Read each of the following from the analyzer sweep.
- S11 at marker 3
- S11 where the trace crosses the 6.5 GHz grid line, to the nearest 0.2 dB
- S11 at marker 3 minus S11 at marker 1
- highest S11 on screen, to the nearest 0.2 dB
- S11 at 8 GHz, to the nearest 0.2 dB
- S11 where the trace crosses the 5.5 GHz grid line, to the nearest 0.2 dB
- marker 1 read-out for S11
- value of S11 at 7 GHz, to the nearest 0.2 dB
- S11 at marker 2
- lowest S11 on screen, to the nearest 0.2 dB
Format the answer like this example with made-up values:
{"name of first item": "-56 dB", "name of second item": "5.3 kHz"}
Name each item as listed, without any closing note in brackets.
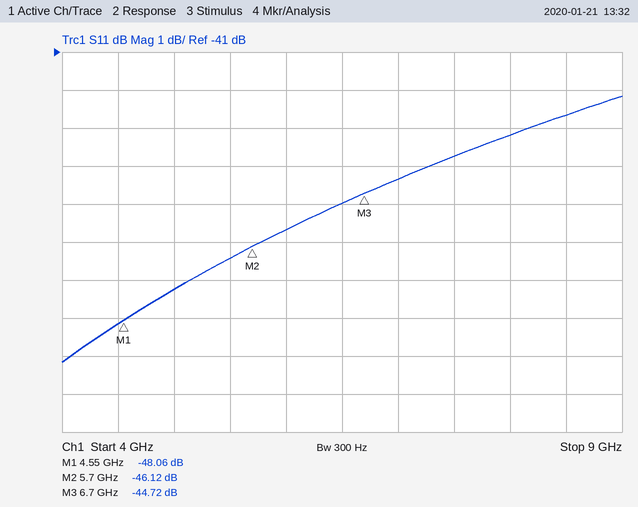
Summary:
{"S11 at marker 3": "-44.72 dB", "S11 where the trace crosses the 6.5 GHz grid line, to the nearest 0.2 dB": "-45.0 dB", "S11 at marker 3 minus S11 at marker 1": "3.34 dB", "highest S11 on screen, to the nearest 0.2 dB": "-42.2 dB", "S11 at 8 GHz, to the nearest 0.2 dB": "-43.2 dB", "S11 where the trace crosses the 5.5 GHz grid line, to the nearest 0.2 dB": "-46.4 dB", "marker 1 read-out for S11": "-48.06 dB", "value of S11 at 7 GHz, to the nearest 0.2 dB": "-44.4 dB", "S11 at marker 2": "-46.12 dB", "lowest S11 on screen, to the nearest 0.2 dB": "-49.2 dB"}
